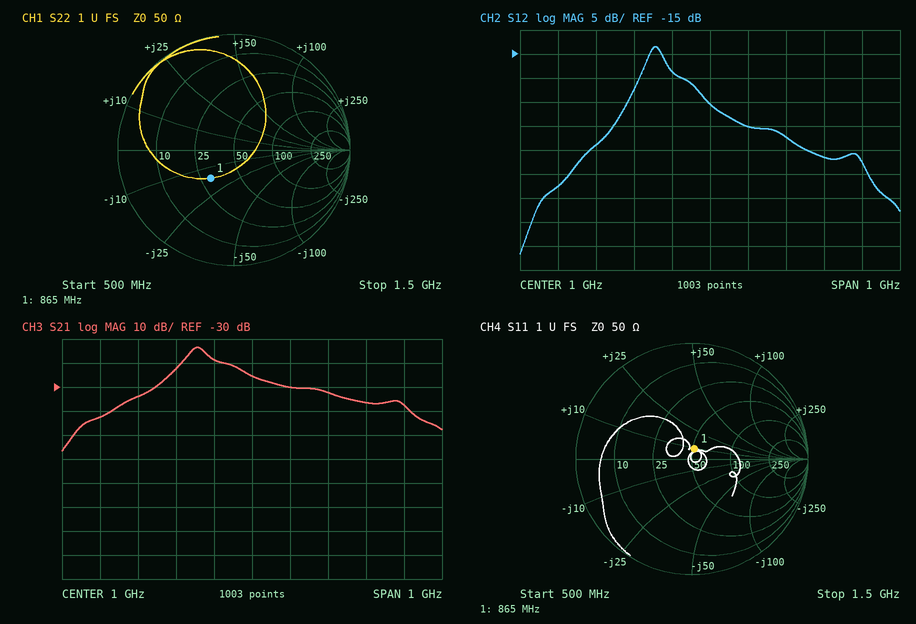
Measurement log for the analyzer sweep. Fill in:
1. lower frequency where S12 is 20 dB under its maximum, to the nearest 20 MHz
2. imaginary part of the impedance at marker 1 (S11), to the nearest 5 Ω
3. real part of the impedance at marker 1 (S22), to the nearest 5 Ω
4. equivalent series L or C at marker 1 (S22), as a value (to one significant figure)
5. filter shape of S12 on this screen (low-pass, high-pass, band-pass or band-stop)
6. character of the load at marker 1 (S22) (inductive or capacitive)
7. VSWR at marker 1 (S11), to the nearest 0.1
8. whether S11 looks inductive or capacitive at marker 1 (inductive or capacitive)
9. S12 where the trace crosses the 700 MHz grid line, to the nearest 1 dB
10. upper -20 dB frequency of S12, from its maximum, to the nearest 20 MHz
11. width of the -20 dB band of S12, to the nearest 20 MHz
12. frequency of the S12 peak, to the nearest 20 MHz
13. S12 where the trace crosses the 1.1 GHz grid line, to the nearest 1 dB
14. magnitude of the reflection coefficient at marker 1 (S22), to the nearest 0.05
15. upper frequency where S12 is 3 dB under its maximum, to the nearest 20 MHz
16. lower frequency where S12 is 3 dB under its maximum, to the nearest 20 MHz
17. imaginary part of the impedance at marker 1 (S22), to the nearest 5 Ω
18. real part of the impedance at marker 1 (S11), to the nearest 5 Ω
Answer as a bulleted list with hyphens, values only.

- 700 MHz
- +10 Ω
- 30 Ω
- 10 pF
- band-pass
- capacitive
- 1.2
- inductive
- -34 dB
- 1.22 GHz
- 520 MHz
- 860 MHz
- -30 dB
- 0.30
- 880 MHz
- 840 MHz
- -15 Ω
- 50 Ω
